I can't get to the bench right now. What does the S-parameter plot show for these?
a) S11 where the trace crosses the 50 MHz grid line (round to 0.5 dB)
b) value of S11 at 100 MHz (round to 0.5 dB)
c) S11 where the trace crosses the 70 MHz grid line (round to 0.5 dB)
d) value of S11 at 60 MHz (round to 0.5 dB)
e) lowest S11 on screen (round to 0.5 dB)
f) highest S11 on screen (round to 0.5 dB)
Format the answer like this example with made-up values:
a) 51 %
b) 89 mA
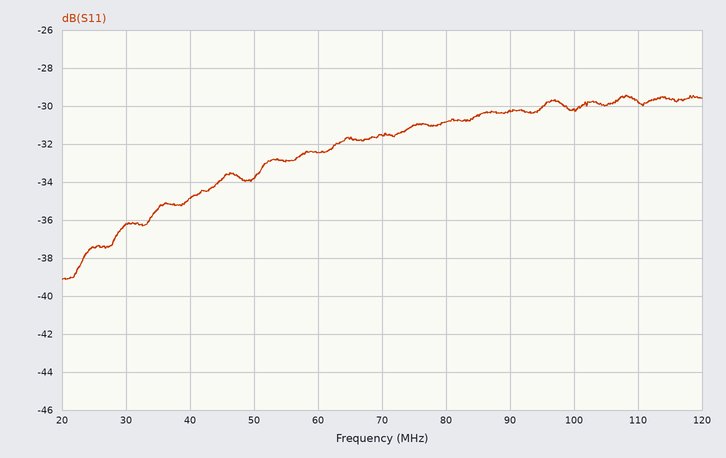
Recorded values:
a) -34.0 dB
b) -30.0 dB
c) -31.5 dB
d) -32.5 dB
e) -39.0 dB
f) -29.5 dB
